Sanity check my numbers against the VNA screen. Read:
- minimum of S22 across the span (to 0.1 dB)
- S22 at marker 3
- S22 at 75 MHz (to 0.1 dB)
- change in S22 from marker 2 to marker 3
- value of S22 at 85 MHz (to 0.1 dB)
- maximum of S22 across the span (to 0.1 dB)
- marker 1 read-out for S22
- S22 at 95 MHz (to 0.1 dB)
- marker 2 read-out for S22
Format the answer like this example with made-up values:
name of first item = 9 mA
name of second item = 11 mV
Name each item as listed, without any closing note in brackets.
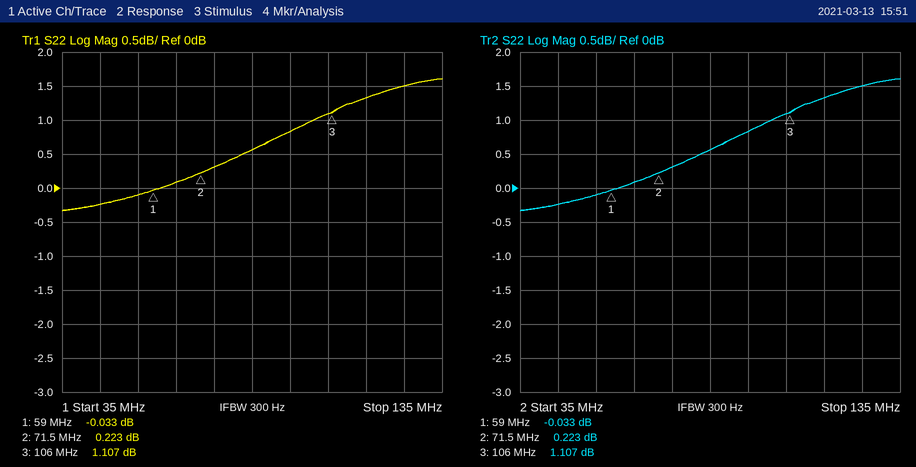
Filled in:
minimum of S22 across the span = -0.3 dB
S22 at marker 3 = 1.107 dB
S22 at 75 MHz = 0.3 dB
change in S22 from marker 2 to marker 3 = 0.884 dB
value of S22 at 85 MHz = 0.6 dB
maximum of S22 across the span = 1.6 dB
marker 1 read-out for S22 = -0.033 dB
S22 at 95 MHz = 0.8 dB
marker 2 read-out for S22 = 0.223 dB
